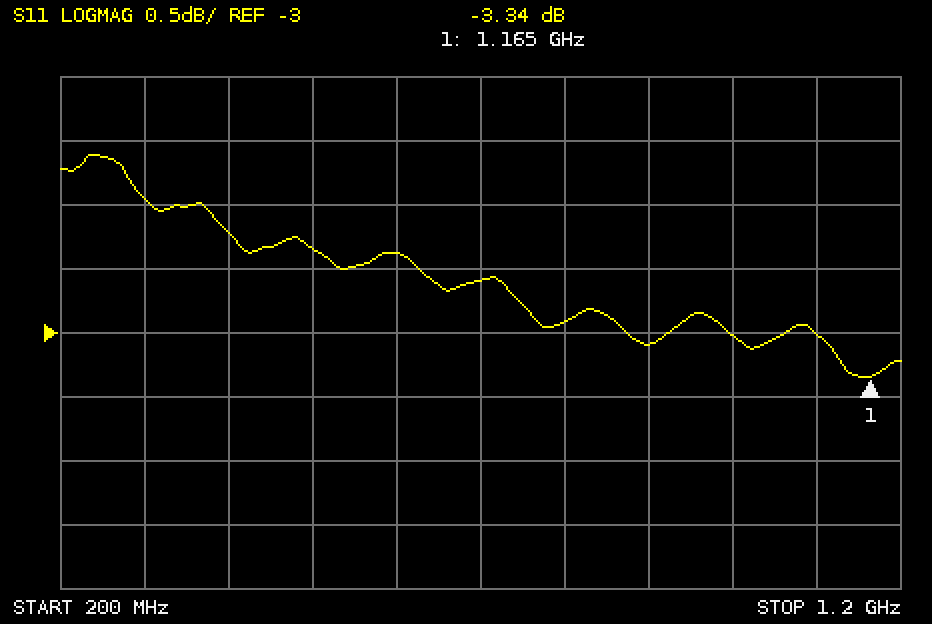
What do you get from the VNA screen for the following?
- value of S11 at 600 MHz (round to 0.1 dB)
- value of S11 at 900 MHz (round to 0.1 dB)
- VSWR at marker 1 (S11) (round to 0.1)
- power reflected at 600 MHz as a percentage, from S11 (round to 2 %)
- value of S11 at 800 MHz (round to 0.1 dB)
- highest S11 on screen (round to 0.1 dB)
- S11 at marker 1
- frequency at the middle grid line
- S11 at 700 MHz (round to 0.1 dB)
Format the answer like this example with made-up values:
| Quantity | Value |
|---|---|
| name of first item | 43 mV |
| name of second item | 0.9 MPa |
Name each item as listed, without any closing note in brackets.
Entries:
| Quantity | Value |
|---|---|
| value of S11 at 600 MHz | -2.4 dB |
| value of S11 at 900 MHz | -3.1 dB |
| VSWR at marker 1 (S11) | 5.3 |
| power reflected at 600 MHz as a percentage, from S11 | 58 % |
| value of S11 at 800 MHz | -2.9 dB |
| highest S11 on screen | -1.6 dB |
| S11 at marker 1 | -3.34 dB |
| frequency at the middle grid line | 700 MHz |
| S11 at 700 MHz | -2.6 dB |
